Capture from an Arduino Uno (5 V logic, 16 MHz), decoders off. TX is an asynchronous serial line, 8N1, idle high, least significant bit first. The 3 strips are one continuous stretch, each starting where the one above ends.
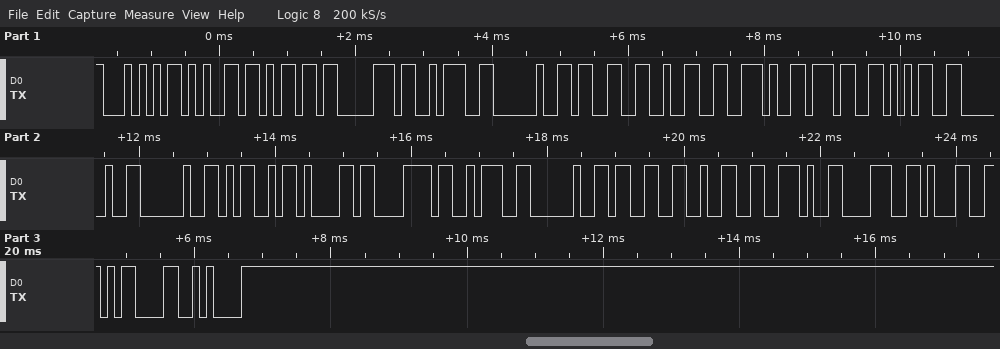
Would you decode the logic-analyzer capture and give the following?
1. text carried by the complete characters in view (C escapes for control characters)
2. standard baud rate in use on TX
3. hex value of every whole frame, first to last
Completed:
"Temp: 32.75  Max: 32.81\r\n"
9600 baud
54 65 6D 70 3A 20 33 32 2E 37 35 20 20 4D 61 78 3A 20 33 32 2E 38 31 0D 0A
